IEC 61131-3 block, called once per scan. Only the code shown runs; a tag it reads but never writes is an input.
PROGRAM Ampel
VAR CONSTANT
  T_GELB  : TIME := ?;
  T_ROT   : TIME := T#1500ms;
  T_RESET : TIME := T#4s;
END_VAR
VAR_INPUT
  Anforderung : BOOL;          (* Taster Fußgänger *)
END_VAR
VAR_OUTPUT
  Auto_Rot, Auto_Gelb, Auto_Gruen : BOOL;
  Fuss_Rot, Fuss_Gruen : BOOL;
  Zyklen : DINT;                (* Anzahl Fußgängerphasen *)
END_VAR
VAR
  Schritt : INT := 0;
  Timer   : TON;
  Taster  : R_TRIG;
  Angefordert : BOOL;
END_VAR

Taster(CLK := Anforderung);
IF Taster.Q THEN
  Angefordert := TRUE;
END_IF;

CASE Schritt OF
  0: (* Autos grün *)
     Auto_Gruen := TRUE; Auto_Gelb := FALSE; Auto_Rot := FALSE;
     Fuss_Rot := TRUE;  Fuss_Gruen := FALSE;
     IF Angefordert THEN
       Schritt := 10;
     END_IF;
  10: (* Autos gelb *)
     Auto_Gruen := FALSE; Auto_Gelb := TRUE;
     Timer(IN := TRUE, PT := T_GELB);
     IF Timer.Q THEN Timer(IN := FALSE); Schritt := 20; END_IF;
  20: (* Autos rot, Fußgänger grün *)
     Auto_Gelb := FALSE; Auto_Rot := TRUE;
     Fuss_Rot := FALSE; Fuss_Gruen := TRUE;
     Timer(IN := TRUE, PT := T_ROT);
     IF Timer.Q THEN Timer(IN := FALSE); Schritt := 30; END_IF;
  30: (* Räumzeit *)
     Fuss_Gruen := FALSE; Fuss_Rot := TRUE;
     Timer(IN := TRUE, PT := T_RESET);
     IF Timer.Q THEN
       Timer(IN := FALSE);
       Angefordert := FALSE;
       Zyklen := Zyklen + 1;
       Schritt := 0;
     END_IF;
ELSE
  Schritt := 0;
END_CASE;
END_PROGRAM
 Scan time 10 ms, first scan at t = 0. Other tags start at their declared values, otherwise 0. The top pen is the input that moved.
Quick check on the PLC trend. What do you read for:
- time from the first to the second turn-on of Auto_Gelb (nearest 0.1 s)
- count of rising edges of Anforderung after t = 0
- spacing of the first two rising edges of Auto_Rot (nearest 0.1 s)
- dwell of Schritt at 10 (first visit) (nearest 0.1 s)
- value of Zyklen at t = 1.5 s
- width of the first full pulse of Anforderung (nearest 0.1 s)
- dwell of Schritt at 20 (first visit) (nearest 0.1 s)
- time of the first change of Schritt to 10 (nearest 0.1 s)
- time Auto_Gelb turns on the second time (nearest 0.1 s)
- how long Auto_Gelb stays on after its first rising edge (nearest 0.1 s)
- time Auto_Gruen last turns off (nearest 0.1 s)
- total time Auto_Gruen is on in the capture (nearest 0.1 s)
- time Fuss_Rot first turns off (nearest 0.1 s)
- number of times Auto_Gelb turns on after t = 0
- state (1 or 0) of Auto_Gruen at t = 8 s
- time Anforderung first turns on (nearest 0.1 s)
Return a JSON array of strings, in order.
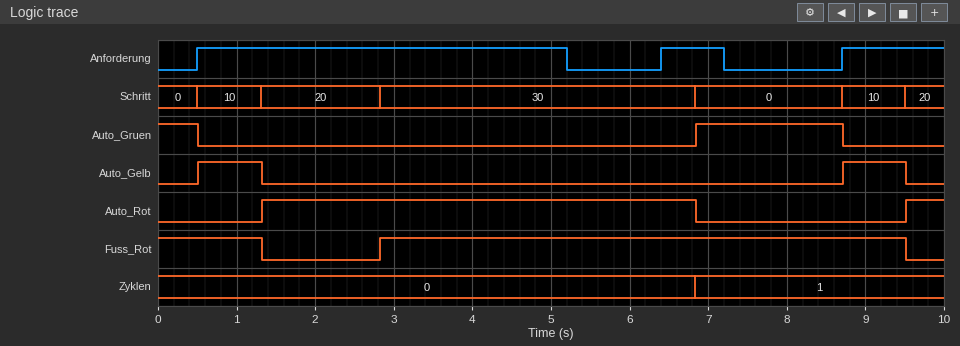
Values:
["8.2 s", "3", "8.2 s", "0.8 s", "0", "4.7 s", "1.5 s", "0.5 s", "8.7 s", "0.8 s", "8.7 s", "2.4 s", "1.3 s", "2", "1", "0.5 s"]
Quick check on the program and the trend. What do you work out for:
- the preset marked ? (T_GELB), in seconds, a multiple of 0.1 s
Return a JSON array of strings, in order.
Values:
["0.8 s"]
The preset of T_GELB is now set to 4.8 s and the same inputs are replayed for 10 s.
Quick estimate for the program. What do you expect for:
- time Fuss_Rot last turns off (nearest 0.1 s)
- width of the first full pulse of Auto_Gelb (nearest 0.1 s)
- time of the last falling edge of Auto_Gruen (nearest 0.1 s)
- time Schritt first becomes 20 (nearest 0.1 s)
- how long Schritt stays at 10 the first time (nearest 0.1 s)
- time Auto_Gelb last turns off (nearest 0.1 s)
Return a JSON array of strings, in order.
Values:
["5.3 s", "4.8 s", "0.5 s", "5.3 s", "4.8 s", "5.3 s"]
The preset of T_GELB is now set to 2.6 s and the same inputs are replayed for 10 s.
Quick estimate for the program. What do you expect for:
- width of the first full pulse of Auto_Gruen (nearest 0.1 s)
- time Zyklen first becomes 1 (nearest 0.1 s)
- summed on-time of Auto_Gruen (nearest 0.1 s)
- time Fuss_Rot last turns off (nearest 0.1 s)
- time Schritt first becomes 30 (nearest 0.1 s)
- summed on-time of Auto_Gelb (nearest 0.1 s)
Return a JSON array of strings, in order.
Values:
["0.1 s", "8.6 s", "0.6 s", "3.1 s", "4.6 s", "3.9 s"]
